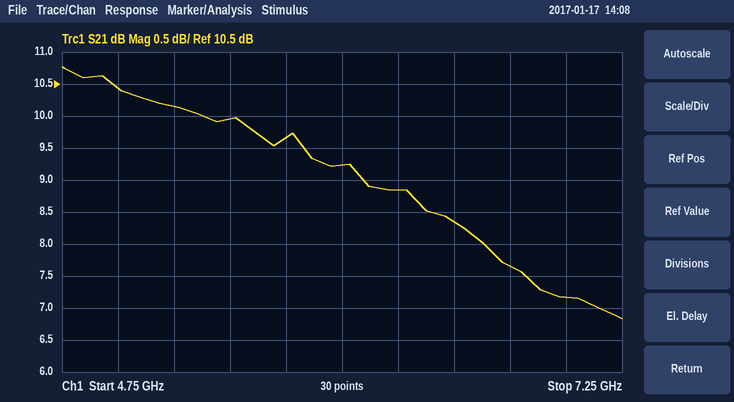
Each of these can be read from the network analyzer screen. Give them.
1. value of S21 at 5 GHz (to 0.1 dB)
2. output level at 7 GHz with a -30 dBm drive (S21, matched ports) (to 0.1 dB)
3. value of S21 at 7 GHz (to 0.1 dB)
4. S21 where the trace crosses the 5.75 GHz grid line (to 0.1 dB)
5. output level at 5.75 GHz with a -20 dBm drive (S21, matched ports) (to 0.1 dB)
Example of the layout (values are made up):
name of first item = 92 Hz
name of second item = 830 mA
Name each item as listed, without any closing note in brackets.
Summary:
value of S21 at 5 GHz = 10.4 dB
output level at 7 GHz with a -30 dBm drive (S21, matched ports) = -22.8 dBm
value of S21 at 7 GHz = 7.2 dB
S21 where the trace crosses the 5.75 GHz grid line = 9.7 dB
output level at 5.75 GHz with a -20 dBm drive (S21, matched ports) = -10.3 dBm
